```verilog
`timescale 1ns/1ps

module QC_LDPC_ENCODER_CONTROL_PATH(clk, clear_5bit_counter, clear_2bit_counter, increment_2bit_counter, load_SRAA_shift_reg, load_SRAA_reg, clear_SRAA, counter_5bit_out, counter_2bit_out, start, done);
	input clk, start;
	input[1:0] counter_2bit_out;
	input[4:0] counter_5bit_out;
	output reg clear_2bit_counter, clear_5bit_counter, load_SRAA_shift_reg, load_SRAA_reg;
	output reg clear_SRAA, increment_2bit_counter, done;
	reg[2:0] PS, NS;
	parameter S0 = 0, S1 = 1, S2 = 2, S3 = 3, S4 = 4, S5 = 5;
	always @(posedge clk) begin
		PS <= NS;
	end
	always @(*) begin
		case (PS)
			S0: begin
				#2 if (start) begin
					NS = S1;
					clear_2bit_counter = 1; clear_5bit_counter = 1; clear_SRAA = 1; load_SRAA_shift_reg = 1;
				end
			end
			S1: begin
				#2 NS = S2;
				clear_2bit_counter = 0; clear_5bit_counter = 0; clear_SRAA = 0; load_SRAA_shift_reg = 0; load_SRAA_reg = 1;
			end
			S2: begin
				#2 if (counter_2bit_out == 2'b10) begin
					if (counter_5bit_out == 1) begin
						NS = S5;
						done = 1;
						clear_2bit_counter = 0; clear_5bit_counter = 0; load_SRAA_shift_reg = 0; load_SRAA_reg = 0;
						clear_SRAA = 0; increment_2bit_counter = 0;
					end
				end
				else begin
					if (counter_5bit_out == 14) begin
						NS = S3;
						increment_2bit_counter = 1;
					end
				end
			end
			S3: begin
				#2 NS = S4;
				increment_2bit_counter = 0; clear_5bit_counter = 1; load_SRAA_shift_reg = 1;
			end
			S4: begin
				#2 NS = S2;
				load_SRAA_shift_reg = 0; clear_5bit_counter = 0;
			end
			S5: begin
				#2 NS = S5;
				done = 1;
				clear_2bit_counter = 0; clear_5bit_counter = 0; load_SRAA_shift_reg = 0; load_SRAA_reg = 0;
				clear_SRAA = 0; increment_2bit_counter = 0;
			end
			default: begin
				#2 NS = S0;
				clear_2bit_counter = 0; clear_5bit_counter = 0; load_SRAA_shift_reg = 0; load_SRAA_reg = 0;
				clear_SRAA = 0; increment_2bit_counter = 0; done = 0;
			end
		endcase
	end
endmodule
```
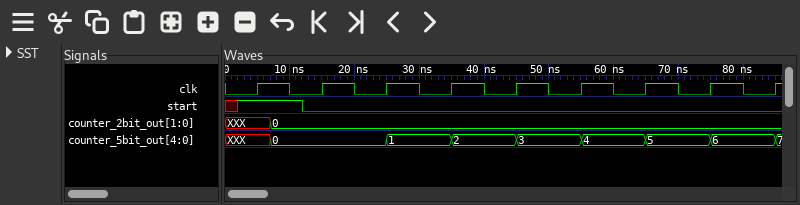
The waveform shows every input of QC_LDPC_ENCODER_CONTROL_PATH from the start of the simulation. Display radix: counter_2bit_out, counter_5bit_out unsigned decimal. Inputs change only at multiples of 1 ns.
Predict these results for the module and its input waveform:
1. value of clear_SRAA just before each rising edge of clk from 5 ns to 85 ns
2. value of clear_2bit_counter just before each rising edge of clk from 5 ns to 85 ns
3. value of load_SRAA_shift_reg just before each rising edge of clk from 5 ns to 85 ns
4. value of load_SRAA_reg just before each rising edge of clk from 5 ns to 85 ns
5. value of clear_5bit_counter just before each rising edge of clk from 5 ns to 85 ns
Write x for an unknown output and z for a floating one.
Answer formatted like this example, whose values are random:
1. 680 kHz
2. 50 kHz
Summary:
1. 0 1 0 0 0 0 0 0 0
2. 0 1 0 0 0 0 0 0 0
3. 0 1 0 0 0 0 0 0 0
4. 0 0 1 1 1 1 1 1 1
5. 0 1 0 0 0 0 0 0 0
